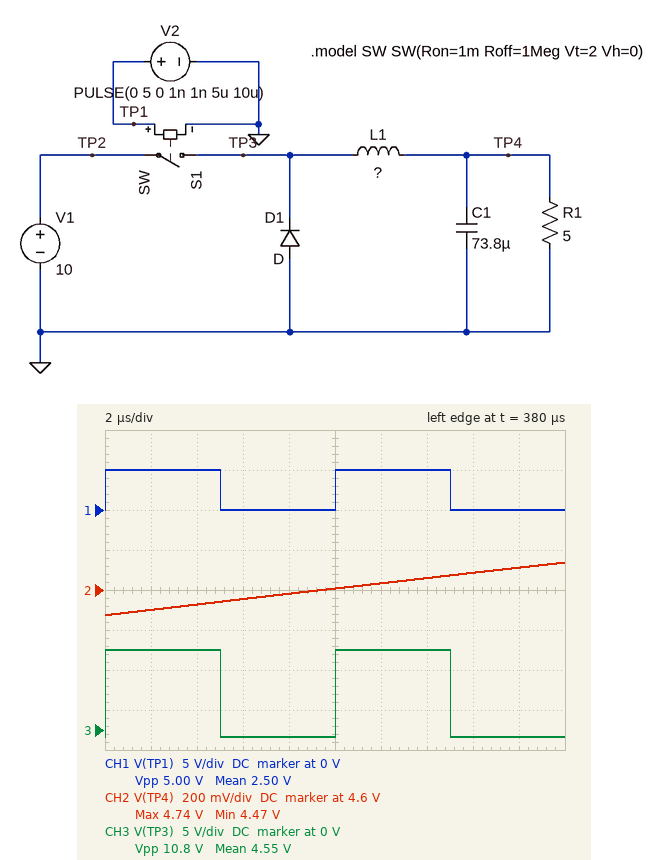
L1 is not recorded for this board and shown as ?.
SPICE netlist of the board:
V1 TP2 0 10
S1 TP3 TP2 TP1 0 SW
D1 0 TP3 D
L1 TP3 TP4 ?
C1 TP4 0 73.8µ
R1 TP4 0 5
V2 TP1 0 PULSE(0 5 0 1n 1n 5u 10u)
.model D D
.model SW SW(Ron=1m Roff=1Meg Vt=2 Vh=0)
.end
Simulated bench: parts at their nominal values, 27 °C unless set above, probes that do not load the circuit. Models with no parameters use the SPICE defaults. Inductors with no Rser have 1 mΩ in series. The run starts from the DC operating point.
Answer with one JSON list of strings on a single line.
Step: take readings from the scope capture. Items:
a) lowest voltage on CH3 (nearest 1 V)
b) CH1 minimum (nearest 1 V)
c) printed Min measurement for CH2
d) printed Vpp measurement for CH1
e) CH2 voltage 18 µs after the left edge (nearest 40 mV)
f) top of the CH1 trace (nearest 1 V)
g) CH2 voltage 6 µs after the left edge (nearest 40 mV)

["-1 V", "0 V", "4.47 V", "5.00 V", "4.72 V", "5 V", "4.56 V"]
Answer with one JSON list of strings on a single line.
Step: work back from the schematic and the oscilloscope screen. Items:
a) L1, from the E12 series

["560 µH"]
